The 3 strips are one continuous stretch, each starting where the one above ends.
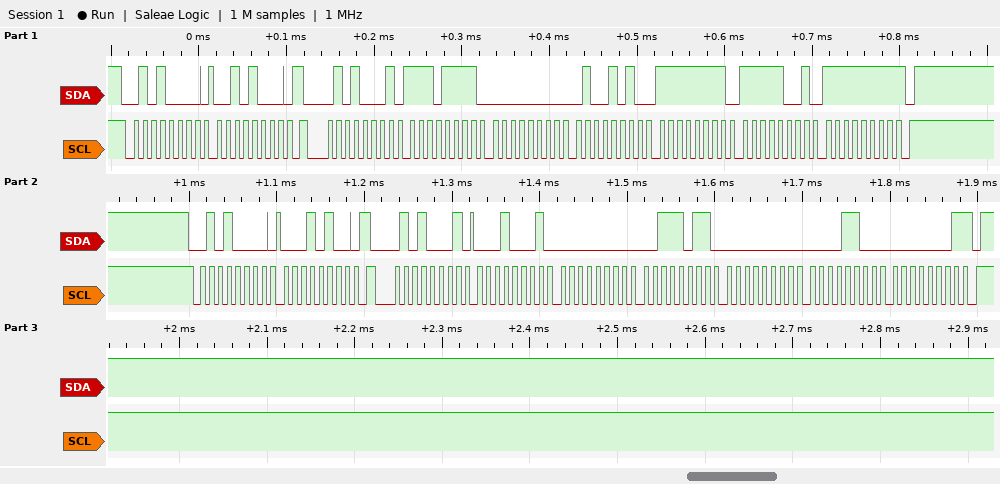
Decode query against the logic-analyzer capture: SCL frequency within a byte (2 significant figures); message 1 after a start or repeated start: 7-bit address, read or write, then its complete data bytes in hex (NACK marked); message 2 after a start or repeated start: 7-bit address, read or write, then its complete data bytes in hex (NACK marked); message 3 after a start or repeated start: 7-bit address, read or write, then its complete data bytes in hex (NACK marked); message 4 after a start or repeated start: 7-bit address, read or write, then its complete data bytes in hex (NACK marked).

100 kHz
0x28 write: 28
0x28 read: EF 00 4A FF F9 FF NACK
0x28 write: 14
0x28 read: 11 00 3B 00 0C 01 NACK
